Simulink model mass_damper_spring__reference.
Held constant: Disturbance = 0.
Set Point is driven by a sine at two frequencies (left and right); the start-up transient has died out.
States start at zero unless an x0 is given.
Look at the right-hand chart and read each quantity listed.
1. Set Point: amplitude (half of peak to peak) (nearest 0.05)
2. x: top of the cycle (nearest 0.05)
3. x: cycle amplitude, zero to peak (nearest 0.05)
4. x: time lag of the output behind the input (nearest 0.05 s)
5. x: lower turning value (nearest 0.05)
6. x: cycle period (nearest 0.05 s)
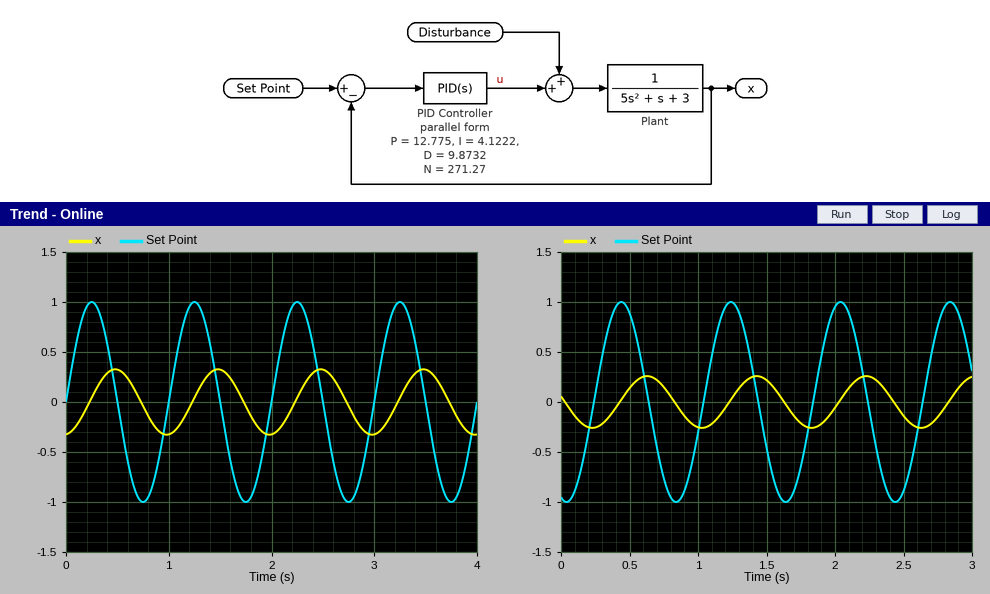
1.00
0.25
0.25
0.20 s
-0.25
0.80 s
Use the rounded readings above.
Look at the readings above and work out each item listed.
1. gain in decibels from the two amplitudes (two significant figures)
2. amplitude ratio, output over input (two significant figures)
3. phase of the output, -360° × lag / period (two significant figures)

-12 dB
0.25
-90°
